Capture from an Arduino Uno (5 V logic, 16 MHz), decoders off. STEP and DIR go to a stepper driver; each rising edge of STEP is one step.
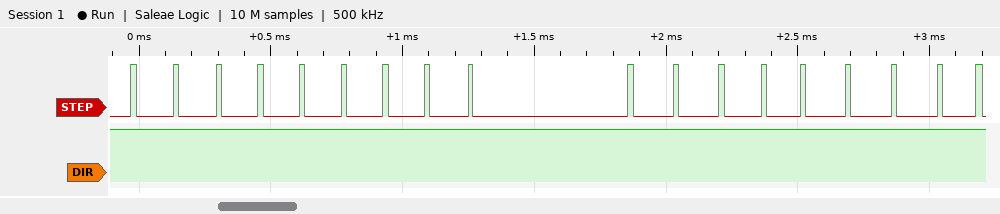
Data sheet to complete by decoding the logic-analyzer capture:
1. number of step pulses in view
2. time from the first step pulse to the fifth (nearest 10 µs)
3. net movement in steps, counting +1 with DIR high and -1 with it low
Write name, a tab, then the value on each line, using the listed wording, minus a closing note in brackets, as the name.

number of step pulses in view	18
time from the first step pulse to the fifth	640 µs
net movement in steps, counting +1 with DIR high and -1 with it low	+18
